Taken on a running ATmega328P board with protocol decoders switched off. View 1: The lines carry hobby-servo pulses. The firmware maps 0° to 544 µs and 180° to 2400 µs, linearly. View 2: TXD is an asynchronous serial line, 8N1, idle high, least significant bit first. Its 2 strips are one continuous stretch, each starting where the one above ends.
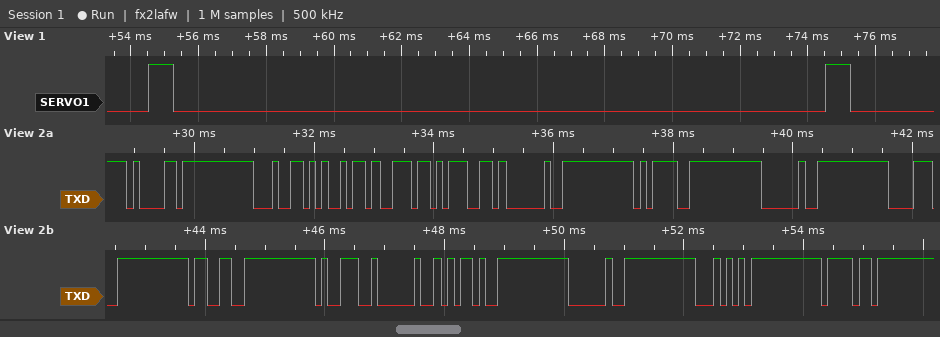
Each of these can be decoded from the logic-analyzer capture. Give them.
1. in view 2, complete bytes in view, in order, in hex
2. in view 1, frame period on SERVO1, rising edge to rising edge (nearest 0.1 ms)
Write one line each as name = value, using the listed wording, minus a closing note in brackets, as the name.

in view 2, complete bytes in view, in order, in hex = 61 64 69 6E 67 20 3D 20 38 33 39 20 2D 20 54 6F
in view 1, frame period on SERVO1, rising edge to rising edge = 20.0 ms
